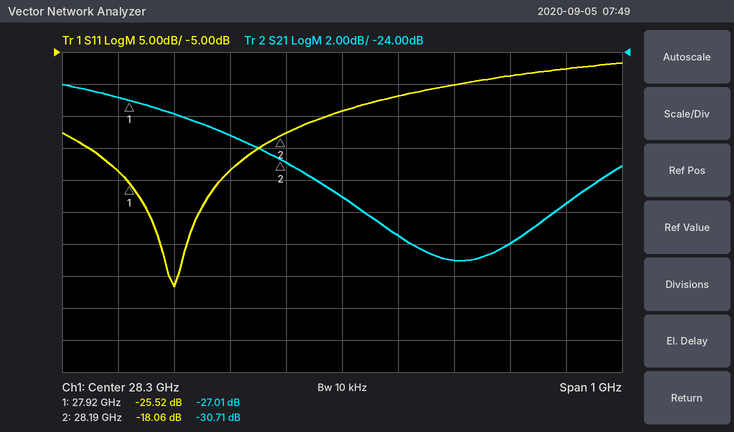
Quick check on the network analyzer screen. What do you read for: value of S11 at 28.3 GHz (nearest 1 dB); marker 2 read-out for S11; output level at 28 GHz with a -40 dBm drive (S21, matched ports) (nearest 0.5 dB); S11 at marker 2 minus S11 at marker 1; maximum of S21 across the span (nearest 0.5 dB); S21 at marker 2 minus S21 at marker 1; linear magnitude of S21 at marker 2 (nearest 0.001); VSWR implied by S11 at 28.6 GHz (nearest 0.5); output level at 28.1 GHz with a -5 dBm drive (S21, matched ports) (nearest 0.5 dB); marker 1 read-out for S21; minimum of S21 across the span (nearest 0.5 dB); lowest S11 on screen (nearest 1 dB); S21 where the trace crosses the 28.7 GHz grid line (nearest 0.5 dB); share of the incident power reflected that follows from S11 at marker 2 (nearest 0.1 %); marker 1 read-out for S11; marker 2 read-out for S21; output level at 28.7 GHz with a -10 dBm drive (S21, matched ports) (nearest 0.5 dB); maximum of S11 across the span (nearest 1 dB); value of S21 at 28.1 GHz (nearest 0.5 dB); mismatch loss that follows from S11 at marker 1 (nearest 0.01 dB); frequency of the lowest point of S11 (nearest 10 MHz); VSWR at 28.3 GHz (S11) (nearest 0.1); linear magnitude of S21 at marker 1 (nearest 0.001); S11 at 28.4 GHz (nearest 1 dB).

-14 dB
-18.06 dB
-68.0 dBm
7.46 dB
-26.0 dB
-3.70 dB
0.029
2.0
-34.0 dBm
-27.01 dB
-37.0 dB
-42 dB
-33.5 dB
1.6 %
-25.52 dB
-30.71 dB
-43.5 dBm
-7 dB
-29.0 dB
0.01 dB
28.00 GHz
1.5
0.045
-12 dB
